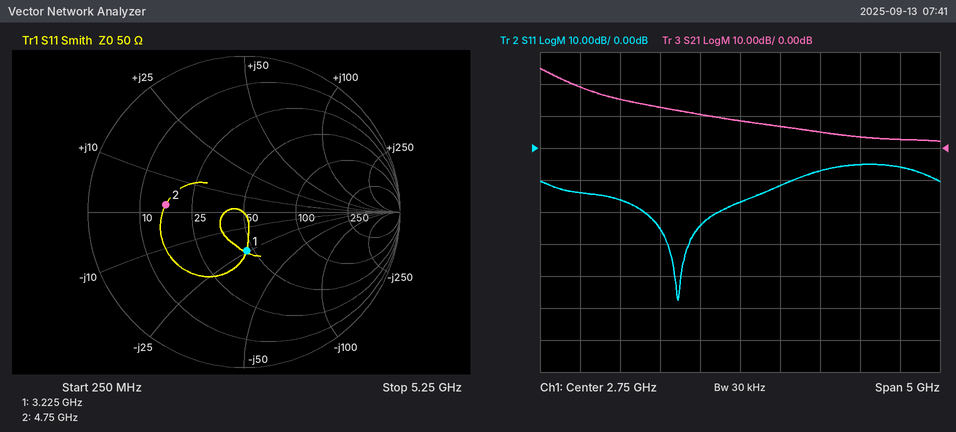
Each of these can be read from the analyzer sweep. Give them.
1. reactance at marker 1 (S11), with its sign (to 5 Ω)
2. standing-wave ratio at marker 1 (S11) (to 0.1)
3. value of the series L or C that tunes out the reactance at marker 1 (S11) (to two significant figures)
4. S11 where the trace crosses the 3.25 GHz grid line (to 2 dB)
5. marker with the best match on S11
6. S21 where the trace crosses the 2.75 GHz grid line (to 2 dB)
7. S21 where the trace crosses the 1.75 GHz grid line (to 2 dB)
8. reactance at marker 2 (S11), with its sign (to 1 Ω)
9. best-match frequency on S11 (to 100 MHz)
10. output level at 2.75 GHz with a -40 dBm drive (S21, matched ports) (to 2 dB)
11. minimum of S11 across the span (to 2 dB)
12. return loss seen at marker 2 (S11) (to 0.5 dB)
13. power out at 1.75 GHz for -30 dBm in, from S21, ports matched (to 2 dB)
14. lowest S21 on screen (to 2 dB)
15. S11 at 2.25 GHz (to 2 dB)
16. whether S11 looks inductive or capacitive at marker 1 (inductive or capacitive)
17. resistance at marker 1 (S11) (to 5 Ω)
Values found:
-25 Ω
1.7
1.2 nH
-12 dB
marker 1
8 dB
12 dB
+2 Ω
2.0 GHz
-32 dBm
-48 dB
6.0 dB
-18 dBm
2 dB
-24 dB
capacitive
45 Ω
